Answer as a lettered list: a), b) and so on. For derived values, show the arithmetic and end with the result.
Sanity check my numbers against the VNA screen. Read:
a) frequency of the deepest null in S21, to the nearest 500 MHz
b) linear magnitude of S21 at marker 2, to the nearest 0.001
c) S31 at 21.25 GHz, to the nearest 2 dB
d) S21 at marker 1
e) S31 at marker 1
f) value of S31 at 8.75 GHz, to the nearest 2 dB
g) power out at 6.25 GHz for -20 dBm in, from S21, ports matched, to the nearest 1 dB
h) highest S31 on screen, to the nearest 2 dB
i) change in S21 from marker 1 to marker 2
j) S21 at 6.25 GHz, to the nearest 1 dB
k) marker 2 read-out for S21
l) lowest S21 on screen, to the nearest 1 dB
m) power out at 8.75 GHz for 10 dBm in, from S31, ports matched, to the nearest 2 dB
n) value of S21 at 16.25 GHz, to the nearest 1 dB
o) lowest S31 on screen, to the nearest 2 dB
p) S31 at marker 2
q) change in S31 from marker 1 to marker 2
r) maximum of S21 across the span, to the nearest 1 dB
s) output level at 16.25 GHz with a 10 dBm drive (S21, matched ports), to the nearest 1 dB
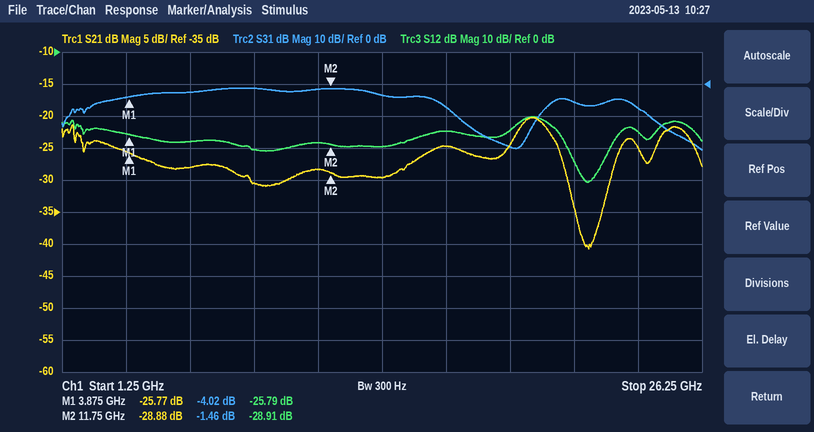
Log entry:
a) 22.0 GHz
b) 10^(-28.88/20) ≈ 0.036
c) -6 dB
d) -25.77 dB
e) -4.02 dB
f) -2 dB
g) -20 dBm + (-28 dB) = -48 dBm
h) -2 dB
i) -28.88 − (-25.77) = -3.11 dB
j) -28 dB
k) -28.88 dB
l) -41 dB
m) 10 dBm + (-2 dB) = 8 dBm
n) -25 dB
o) -20 dB
p) -1.46 dB
q) -1.46 − (-4.02) = 2.56 dB
r) -20 dB
s) 10 dBm + (-25 dB) = -15 dBm
